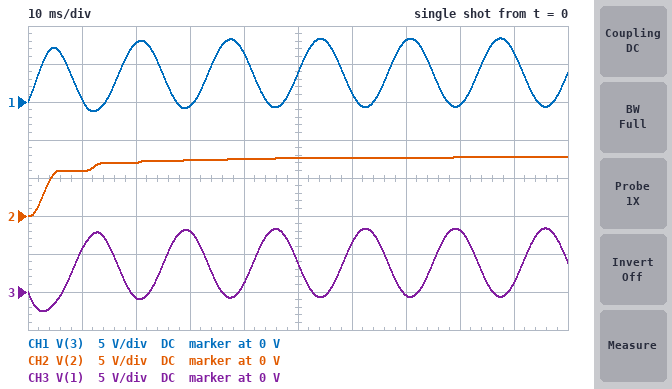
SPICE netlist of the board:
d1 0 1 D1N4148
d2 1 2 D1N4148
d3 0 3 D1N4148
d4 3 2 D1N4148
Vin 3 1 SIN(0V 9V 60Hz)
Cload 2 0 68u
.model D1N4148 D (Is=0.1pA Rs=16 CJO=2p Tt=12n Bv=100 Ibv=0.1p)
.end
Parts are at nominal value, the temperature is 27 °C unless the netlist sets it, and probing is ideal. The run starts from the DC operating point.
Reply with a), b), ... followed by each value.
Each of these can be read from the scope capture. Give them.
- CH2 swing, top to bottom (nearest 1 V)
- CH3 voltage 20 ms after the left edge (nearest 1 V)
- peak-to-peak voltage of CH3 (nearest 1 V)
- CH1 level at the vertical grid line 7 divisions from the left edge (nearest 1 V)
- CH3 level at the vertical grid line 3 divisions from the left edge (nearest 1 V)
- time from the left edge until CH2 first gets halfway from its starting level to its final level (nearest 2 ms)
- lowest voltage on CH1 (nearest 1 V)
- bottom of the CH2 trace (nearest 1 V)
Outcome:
a) 8 V
b) -1 V
c) 11 V
d) 8 V
e) 8 V
f) 4 ms
g) -1 V
h) 0 V
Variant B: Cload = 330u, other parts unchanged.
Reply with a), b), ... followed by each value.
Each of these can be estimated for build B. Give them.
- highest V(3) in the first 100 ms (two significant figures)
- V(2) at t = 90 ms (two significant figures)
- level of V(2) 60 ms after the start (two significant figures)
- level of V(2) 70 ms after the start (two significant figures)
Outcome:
a) 8.0 V
b) 7.0 V
c) 6.5 V
d) 6.7 V
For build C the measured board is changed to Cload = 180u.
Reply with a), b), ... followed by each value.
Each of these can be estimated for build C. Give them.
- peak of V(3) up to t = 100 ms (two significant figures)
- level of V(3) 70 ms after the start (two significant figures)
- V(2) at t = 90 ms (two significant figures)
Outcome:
a) 8.2 V
b) 7.9 V
c) 7.4 V
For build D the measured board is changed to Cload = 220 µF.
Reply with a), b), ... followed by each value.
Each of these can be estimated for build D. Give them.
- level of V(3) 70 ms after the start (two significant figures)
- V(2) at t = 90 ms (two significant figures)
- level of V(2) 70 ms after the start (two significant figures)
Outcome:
a) 7.8 V
b) 7.3 V
c) 7.1 V
